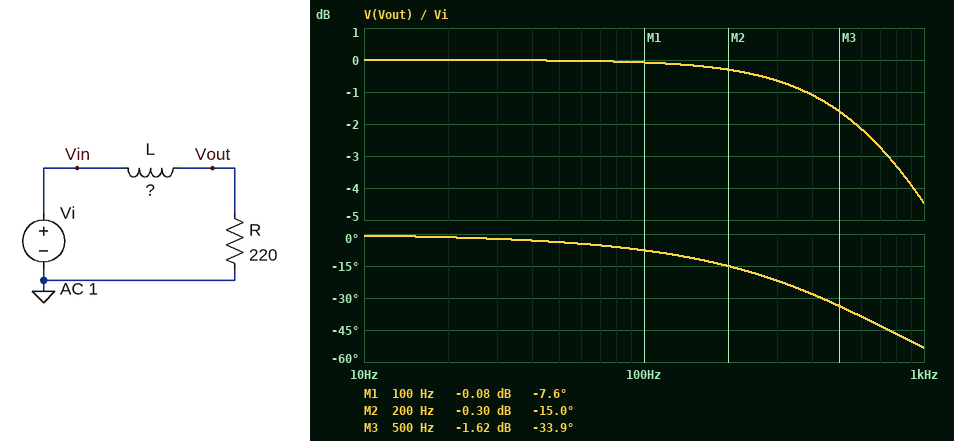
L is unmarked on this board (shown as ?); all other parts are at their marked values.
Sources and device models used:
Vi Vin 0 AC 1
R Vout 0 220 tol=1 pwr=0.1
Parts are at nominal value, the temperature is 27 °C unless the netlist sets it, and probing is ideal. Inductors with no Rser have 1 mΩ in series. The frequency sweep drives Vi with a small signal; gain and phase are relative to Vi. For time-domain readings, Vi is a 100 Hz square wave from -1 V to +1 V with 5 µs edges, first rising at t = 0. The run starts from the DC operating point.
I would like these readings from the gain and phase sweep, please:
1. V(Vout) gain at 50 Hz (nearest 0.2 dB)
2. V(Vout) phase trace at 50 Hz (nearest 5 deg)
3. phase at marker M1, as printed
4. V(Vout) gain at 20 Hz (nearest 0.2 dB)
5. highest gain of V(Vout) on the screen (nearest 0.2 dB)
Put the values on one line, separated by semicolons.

0 dB; -5 deg; -7.6 deg; 0 dB; 0 dB
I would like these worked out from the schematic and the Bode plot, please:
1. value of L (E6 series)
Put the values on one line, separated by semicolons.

47 mH
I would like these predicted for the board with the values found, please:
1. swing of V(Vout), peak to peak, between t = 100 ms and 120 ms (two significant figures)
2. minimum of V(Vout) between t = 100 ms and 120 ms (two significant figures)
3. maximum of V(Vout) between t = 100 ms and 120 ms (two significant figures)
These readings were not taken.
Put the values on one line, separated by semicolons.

2.0 V; -1.0 V; 1.0 V
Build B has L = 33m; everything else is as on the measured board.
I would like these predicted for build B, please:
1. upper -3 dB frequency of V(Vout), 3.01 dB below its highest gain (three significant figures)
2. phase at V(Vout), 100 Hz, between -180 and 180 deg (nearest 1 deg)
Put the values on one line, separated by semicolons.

1.06 kHz; -5 deg
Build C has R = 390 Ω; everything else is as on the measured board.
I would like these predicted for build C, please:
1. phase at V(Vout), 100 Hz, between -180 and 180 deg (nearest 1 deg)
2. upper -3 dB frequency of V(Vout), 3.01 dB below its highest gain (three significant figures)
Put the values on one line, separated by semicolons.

-4 deg; 1.32 kHz
